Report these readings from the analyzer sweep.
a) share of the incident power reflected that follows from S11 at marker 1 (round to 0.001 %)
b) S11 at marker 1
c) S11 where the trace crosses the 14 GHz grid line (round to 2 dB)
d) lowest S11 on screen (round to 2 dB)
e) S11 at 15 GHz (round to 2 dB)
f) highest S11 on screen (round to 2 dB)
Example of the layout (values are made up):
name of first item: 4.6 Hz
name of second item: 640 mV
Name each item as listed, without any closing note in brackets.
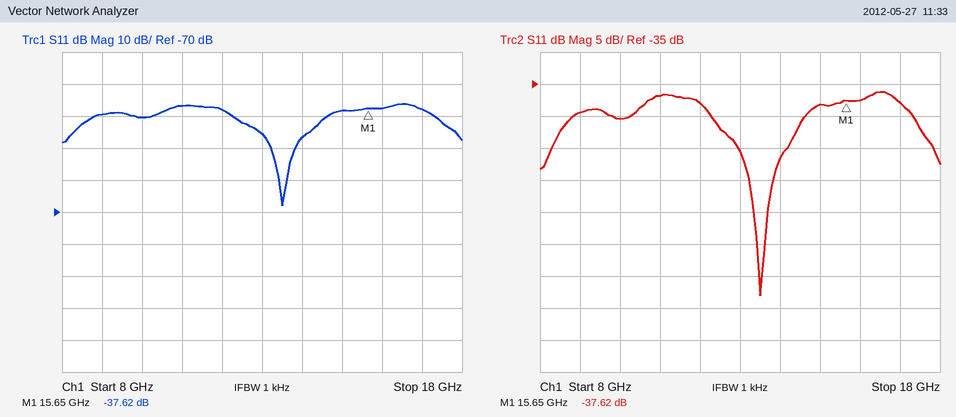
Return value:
share of the incident power reflected that follows from S11 at marker 1: 0.017 %
S11 at marker 1: -37.62 dB
S11 where the trace crosses the 14 GHz grid line: -46 dB
lowest S11 on screen: -68 dB
S11 at 15 GHz: -38 dB
highest S11 on screen: -36 dB
